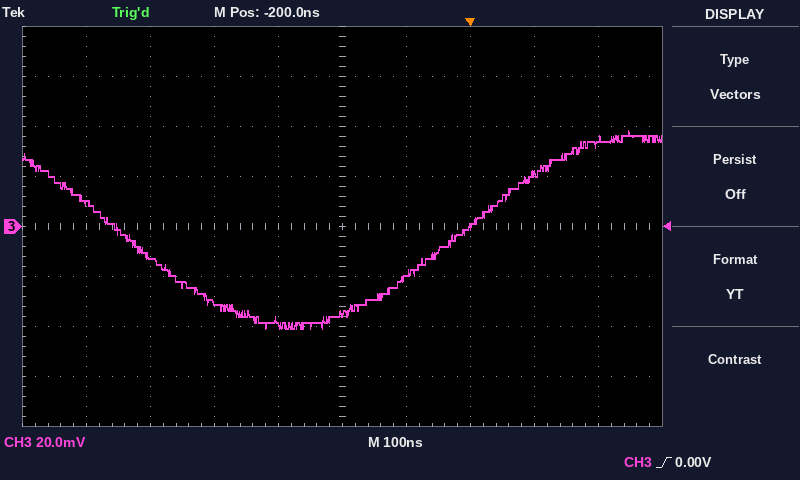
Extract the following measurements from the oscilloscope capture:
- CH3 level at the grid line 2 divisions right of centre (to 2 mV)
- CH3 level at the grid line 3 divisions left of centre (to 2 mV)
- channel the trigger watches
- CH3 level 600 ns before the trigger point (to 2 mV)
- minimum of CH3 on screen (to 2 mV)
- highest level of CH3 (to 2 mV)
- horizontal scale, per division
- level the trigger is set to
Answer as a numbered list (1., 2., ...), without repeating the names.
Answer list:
1. 0 mV
2. -12 mV
3. CH3
4. 10 mV
5. -40 mV
6. 38 mV
7. 100 ns
8. 0.00 V
